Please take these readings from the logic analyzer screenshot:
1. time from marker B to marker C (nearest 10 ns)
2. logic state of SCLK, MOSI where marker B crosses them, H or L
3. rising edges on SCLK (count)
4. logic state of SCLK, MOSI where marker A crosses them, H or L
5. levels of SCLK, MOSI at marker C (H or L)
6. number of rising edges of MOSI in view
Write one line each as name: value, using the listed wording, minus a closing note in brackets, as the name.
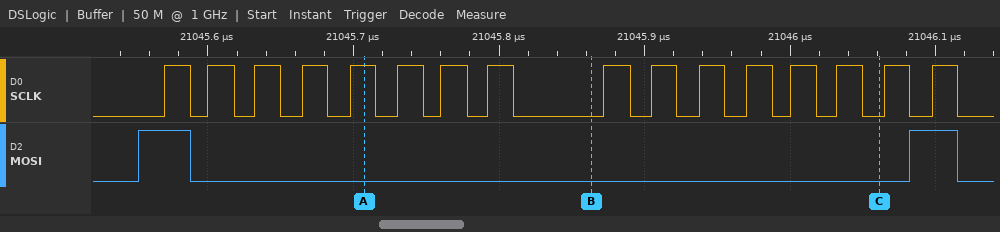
time from marker B to marker C: 200 ns
logic state of SCLK, MOSI where marker B crosses them, H or L: SCLK=L, MOSI=L
rising edges on SCLK: 16
logic state of SCLK, MOSI where marker A crosses them, H or L: SCLK=H, MOSI=L
levels of SCLK, MOSI at marker C: SCLK=L, MOSI=L
number of rising edges of MOSI in view: 2
